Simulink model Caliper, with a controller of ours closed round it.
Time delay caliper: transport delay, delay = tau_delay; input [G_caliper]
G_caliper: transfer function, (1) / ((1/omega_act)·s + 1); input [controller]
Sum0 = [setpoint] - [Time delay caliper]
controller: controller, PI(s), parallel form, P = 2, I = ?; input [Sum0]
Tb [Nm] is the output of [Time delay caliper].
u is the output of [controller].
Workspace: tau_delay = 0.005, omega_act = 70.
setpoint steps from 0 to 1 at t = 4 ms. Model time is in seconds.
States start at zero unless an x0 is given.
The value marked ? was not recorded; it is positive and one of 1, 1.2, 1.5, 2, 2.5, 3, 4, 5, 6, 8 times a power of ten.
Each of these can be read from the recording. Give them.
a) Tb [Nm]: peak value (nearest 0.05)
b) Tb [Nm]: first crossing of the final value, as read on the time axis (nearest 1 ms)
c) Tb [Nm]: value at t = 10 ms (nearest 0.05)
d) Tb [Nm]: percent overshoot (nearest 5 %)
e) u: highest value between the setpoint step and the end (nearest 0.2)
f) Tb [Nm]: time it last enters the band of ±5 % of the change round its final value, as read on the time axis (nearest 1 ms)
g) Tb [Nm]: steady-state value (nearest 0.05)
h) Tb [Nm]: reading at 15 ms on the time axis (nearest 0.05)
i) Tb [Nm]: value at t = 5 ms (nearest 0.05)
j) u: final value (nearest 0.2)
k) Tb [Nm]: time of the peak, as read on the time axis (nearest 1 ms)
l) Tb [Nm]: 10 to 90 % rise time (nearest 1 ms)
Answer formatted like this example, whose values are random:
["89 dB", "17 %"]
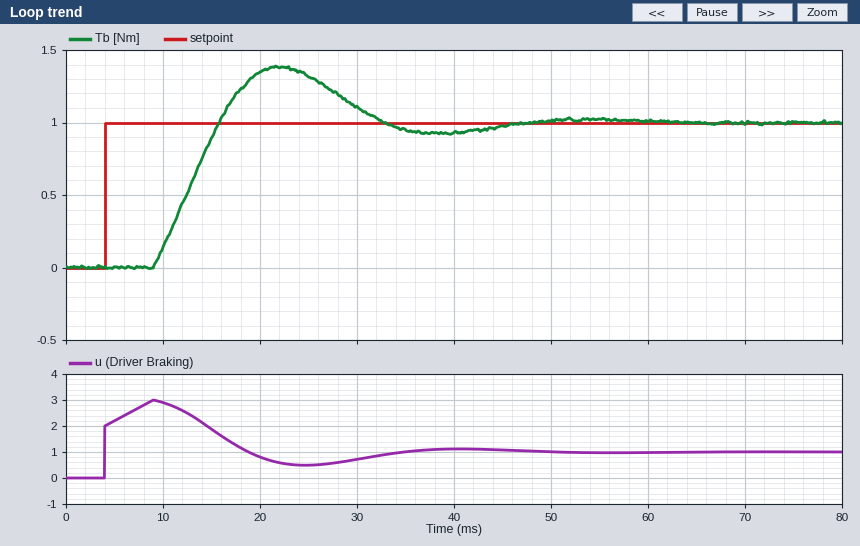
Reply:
["1.40", "16 ms", "0.15", "40 %", "3.0", "43 ms", "1.00", "0.90", "0.00", "1.0", "22 ms", "5 ms"]
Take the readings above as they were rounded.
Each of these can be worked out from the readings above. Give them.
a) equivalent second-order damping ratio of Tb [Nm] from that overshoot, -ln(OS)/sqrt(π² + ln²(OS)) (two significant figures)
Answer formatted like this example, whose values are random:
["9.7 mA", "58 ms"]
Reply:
["0.28"]
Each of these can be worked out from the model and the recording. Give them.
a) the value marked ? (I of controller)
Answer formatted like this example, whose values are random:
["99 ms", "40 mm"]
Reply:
["200"]
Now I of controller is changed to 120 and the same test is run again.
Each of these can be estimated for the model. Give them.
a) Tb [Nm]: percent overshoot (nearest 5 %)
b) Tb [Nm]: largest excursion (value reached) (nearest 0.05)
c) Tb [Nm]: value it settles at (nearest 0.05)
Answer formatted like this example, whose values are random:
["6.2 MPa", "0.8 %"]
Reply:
["15 %", "1.15", "1.00"]
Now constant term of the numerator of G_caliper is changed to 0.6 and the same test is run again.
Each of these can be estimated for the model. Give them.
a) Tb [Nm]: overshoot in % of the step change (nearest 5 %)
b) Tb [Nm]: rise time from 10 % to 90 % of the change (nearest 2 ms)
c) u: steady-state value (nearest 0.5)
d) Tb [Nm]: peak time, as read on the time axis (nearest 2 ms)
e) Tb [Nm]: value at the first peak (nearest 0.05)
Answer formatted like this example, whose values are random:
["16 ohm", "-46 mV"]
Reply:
["15 %", "10 ms", "1.5", "30 ms", "1.15"]
